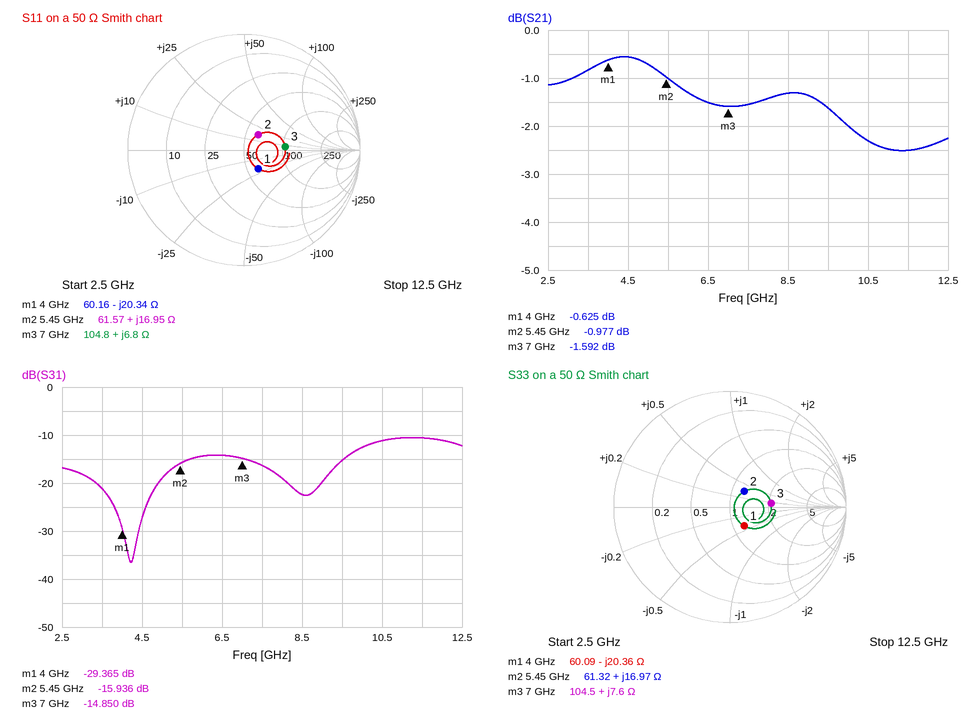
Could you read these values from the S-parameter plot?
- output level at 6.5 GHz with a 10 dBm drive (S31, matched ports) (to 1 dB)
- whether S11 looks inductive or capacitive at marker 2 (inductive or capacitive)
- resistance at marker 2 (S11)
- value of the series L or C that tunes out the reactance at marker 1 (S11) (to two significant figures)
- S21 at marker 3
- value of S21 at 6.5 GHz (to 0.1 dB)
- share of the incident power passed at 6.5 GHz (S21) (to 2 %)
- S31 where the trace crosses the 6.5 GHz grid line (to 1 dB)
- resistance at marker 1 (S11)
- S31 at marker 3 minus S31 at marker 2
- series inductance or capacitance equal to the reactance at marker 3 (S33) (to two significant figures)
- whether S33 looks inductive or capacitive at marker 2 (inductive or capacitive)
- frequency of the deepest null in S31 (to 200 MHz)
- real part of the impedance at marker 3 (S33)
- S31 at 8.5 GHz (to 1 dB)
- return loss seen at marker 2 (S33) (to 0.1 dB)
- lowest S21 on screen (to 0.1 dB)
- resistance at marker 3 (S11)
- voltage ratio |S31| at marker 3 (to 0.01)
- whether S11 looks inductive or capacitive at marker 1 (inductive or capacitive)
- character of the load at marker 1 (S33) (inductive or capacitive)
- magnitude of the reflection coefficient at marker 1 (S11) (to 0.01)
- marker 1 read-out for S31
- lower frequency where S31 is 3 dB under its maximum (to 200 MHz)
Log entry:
-4 dBm
inductive
61.57 Ω
810 pH
-1.592 dB
-1.5 dB
70 %
-14 dB
60.16 Ω
1.086 dB
170 pH
inductive
4.2 GHz
104.5 Ω
-22 dB
14.8 dB
-2.5 dB
104.8 Ω
0.18
capacitive
capacitive
0.20
-29.365 dB
9.8 GHz
